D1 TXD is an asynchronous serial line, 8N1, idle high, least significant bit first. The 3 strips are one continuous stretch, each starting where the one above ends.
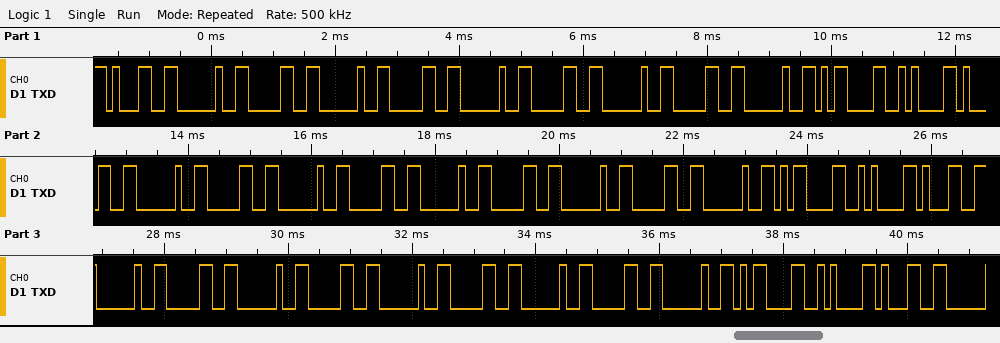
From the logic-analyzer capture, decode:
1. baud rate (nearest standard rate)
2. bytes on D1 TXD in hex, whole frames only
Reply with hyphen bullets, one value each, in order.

- 9600 baud
- 0x31 0x20 0x30 0x20 0x30 0x20 0x30 0x20 0x30 0x20 0x0D 0x0A 0x31 0x20 0x30 0x20 0x30 0x20 0x30 0x20 0x30 0x20 0x0D 0x0A 0x31 0x20 0x30 0x20 0x30 0x20 0x30 0x20 0x30 0x20 0x0D 0x0A 0x31
